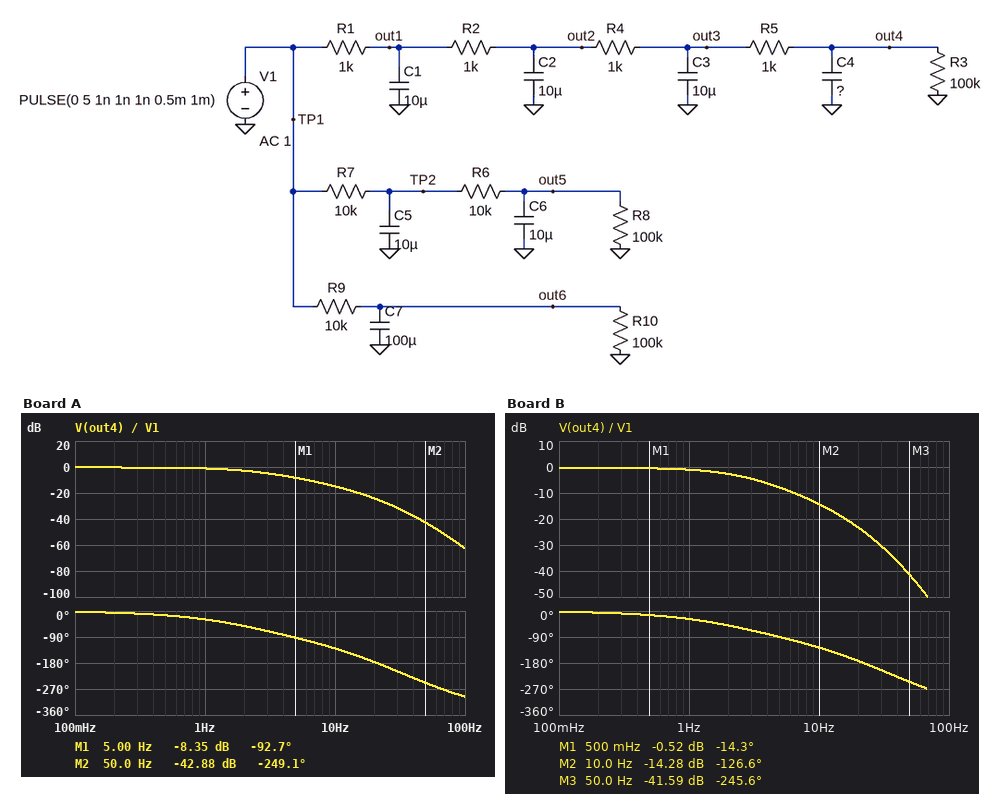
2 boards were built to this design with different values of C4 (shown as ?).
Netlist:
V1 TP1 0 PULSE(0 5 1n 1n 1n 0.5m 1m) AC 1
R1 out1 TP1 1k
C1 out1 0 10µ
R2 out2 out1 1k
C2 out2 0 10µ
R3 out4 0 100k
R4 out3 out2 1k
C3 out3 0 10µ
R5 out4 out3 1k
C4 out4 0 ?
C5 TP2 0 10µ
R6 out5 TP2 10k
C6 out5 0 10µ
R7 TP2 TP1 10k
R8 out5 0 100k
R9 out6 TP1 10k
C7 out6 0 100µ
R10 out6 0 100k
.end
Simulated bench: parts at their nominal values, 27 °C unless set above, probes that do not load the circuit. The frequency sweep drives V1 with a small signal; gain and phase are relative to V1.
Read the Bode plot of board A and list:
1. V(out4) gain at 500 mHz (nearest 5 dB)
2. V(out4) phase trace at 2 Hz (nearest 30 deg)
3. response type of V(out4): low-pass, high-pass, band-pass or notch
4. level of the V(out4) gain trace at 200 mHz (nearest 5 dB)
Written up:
0 dB
-60 deg
low-pass
0 dB
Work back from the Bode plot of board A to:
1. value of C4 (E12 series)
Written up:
6.8 µF
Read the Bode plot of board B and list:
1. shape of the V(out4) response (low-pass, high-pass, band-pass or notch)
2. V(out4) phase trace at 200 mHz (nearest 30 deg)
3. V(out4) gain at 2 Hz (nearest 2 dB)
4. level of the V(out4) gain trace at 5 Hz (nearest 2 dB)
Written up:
low-pass
0 deg
-2 dB
-8 dB
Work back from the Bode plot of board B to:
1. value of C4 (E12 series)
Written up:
5.6 µF
